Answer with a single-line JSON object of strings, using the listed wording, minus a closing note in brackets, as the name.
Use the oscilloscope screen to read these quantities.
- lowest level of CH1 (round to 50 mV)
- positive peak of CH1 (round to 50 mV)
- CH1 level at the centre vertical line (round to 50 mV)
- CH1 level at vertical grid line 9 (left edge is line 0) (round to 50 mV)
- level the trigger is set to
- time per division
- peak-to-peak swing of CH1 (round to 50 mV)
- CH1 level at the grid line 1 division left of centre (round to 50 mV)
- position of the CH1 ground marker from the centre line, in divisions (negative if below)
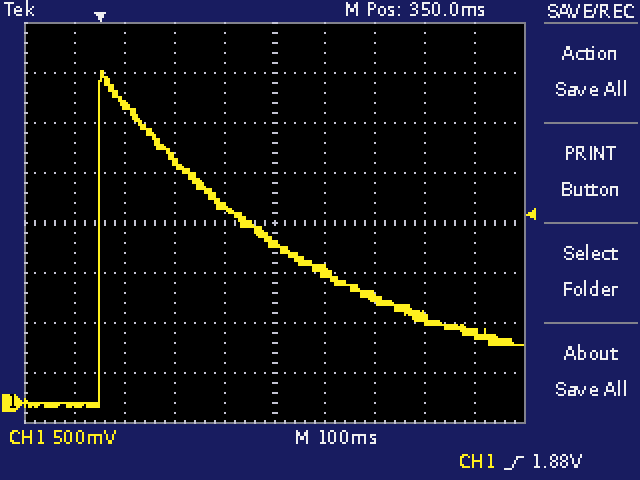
{"lowest level of CH1": "-50 mV", "positive peak of CH1": "3.30 V", "CH1 level at the centre vertical line": "1.60 V", "CH1 level at vertical grid line 9 (left edge is line 0)": "700 mV", "level the trigger is set to": "1.88 V", "time per division": "100 ms", "peak-to-peak swing of CH1": "3.35 V", "CH1 level at the grid line 1 division left of centre": "1.95 V", "position of the CH1 ground marker from the centre line, in divisions": "-3.6 div"}
